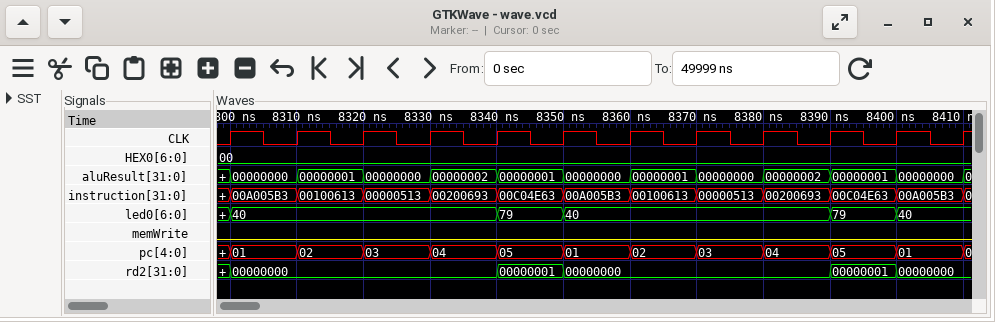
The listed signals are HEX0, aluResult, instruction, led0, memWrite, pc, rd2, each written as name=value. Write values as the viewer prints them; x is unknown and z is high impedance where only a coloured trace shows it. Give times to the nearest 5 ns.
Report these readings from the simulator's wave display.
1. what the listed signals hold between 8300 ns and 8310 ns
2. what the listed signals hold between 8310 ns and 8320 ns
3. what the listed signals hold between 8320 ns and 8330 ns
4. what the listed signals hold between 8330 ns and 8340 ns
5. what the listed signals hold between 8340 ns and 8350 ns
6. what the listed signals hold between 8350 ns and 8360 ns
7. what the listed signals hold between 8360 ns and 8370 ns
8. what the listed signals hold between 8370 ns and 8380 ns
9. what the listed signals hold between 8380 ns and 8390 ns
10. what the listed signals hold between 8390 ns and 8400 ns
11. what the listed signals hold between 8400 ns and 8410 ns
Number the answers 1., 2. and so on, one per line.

1. HEX0=00, aluResult=00000000, instruction=00A005B3, led0=40, memWrite=0, pc=01, rd2=00000000
2. HEX0=00, aluResult=00000001, instruction=00100613, led0=40, memWrite=0, pc=02, rd2=00000000
3. HEX0=00, aluResult=00000000, instruction=00000513, led0=40, memWrite=0, pc=03, rd2=00000000
4. HEX0=00, aluResult=00000002, instruction=00200693, led0=40, memWrite=0, pc=04, rd2=00000000
5. HEX0=00, aluResult=00000001, instruction=00C04E63, led0=79, memWrite=0, pc=05, rd2=00000001
6. HEX0=00, aluResult=00000000, instruction=00A005B3, led0=40, memWrite=0, pc=01, rd2=00000000
7. HEX0=00, aluResult=00000001, instruction=00100613, led0=40, memWrite=0, pc=02, rd2=00000000
8. HEX0=00, aluResult=00000000, instruction=00000513, led0=40, memWrite=0, pc=03, rd2=00000000
9. HEX0=00, aluResult=00000002, instruction=00200693, led0=40, memWrite=0, pc=04, rd2=00000000
10. HEX0=00, aluResult=00000001, instruction=00C04E63, led0=79, memWrite=0, pc=05, rd2=00000001
11. HEX0=00, aluResult=00000000, instruction=00A005B3, led0=40, memWrite=0, pc=01, rd2=00000000
